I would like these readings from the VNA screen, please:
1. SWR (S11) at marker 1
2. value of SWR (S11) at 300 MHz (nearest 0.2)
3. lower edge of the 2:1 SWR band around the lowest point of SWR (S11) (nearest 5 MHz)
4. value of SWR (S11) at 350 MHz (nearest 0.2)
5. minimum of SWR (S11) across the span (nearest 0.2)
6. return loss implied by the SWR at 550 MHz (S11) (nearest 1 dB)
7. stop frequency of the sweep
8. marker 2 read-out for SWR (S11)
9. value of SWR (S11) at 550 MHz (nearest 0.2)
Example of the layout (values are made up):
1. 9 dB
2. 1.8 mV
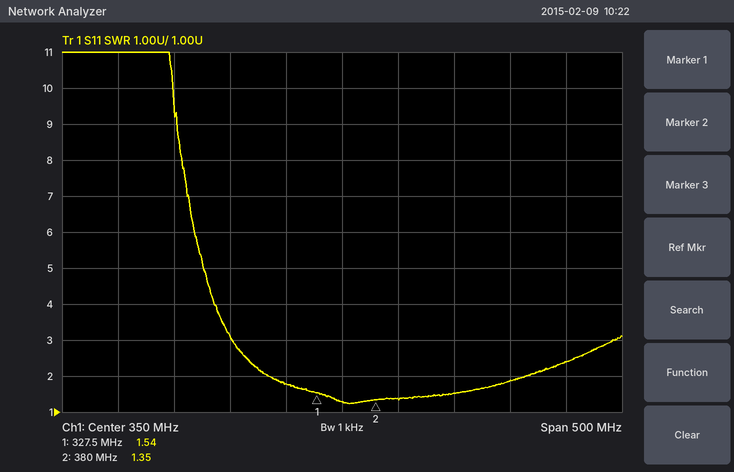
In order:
1. 1.54
2. 1.8
3. 285 MHz
4. 1.2
5. 1.2
6. 8 dB
7. 600 MHz
8. 1.35
9. 2.4
